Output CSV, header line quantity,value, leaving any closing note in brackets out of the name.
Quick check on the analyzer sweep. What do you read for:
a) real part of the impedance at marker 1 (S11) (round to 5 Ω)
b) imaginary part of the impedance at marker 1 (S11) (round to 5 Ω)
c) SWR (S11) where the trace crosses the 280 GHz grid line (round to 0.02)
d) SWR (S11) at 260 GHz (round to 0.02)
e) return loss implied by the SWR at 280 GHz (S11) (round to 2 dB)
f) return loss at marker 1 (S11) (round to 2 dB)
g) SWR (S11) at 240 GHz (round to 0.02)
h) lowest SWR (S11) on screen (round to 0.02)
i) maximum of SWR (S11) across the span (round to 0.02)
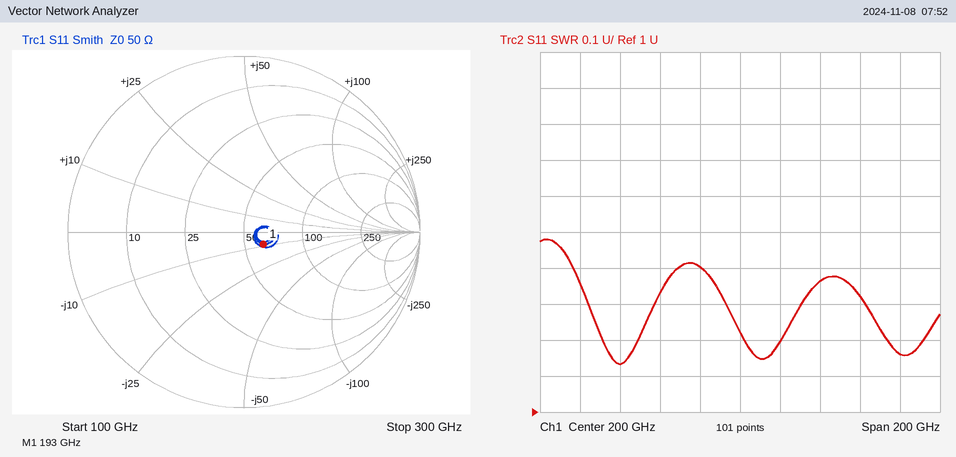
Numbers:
quantity,value
real part of the impedance at marker 1 (S11),60 Ω
imaginary part of the impedance at marker 1 (S11),-10 Ω
SWR (S11) where the trace crosses the 280 GHz grid line,1.16
SWR (S11) at 260 GHz,1.32
return loss implied by the SWR at 280 GHz (S11),22 dB
return loss at marker 1 (S11),18 dB
SWR (S11) at 240 GHz,1.36
lowest SWR (S11) on screen,1.14
maximum of SWR (S11) across the span,1.48
